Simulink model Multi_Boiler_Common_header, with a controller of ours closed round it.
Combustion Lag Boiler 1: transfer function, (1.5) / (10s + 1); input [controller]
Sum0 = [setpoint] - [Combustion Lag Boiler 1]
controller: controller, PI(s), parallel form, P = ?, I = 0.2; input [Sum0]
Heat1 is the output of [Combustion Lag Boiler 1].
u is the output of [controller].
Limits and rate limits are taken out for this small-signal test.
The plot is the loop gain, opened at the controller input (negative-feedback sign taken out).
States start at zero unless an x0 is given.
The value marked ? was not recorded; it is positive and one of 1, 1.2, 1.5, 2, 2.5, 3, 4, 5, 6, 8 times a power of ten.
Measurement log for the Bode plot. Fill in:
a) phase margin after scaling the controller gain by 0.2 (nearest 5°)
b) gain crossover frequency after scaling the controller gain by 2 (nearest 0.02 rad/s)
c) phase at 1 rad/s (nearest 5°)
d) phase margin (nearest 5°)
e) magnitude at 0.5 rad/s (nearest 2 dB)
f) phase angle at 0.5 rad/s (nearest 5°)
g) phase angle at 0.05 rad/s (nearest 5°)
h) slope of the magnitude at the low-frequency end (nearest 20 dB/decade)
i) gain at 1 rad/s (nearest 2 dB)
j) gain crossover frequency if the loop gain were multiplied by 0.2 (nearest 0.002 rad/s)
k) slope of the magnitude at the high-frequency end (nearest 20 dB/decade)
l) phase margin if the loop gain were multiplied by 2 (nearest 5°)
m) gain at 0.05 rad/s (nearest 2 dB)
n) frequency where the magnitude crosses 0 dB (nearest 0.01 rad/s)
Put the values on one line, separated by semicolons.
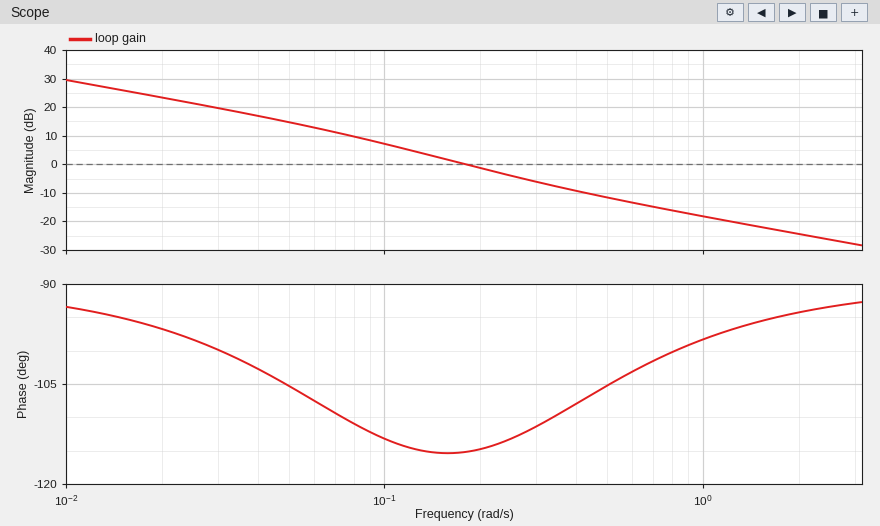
75°; 0.30 rad/s; -100°; 65°; -12 dB; -105°; -105°; -20 dB/decade; -18 dB; 0.054 rad/s; -20 dB/decade; 70°; 14 dB; 0.18 rad/s
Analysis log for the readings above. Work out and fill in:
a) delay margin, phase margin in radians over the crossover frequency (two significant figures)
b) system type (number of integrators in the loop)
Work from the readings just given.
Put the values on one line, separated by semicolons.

6.3 s; 1
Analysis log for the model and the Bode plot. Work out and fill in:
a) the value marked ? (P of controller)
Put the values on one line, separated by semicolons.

0.8
